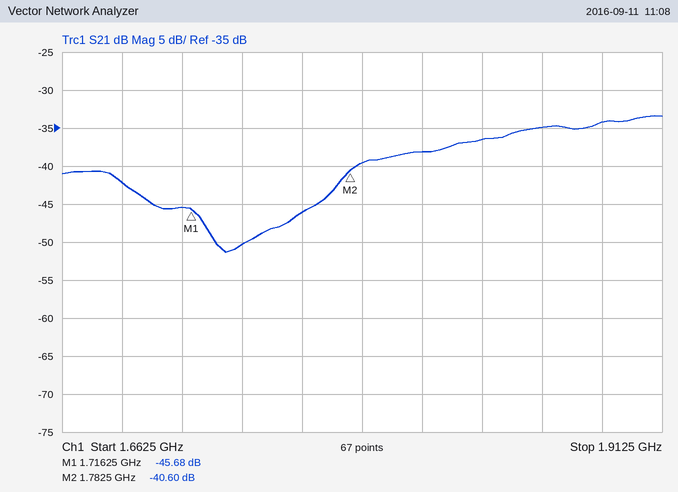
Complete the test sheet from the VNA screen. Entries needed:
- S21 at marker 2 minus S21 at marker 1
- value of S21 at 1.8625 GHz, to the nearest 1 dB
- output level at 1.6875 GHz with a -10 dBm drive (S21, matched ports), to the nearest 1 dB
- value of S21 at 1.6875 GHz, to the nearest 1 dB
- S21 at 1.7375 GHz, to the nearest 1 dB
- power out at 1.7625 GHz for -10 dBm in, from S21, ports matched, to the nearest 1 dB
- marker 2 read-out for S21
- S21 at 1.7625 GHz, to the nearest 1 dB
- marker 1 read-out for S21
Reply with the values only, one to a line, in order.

5.08 dB
-35 dB
-52 dBm
-42 dB
-50 dB
-56 dBm
-40.60 dB
-46 dB
-45.68 dB
